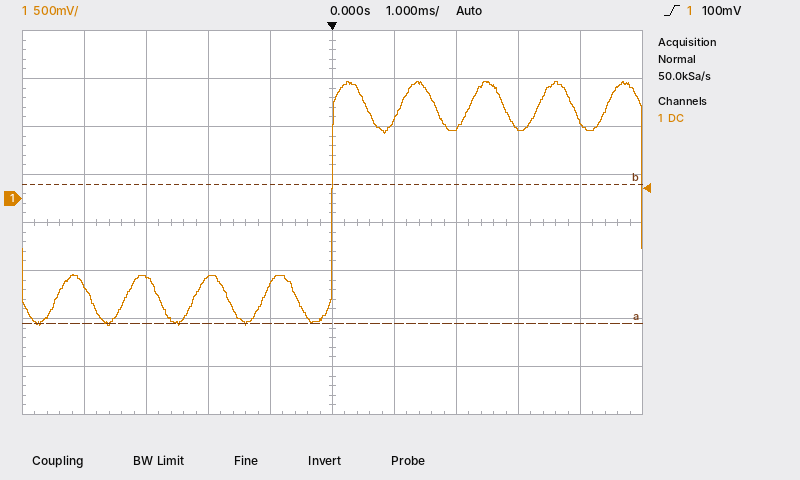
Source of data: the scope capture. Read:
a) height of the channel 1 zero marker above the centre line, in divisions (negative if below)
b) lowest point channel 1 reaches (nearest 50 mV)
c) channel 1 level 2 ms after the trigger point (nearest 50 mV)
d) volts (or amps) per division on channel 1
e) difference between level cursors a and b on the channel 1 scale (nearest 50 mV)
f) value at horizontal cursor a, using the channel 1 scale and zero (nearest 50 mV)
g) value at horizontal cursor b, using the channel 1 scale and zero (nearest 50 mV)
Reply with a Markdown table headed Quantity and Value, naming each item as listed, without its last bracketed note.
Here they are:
| Quantity | Value |
|---|---|
| height of the channel 1 zero marker above the centre line, in divisions | +0.5 div |
| lowest point channel 1 reaches | -1.30 V |
| channel 1 level 2 ms after the trigger point | 750 mV |
| volts (or amps) per division on channel 1 | 500 mV |
| difference between level cursors a and b on the channel 1 scale | 1.45 V |
| value at horizontal cursor a, using the channel 1 scale and zero | -1.30 V |
| value at horizontal cursor b, using the channel 1 scale and zero | 150 mV |
